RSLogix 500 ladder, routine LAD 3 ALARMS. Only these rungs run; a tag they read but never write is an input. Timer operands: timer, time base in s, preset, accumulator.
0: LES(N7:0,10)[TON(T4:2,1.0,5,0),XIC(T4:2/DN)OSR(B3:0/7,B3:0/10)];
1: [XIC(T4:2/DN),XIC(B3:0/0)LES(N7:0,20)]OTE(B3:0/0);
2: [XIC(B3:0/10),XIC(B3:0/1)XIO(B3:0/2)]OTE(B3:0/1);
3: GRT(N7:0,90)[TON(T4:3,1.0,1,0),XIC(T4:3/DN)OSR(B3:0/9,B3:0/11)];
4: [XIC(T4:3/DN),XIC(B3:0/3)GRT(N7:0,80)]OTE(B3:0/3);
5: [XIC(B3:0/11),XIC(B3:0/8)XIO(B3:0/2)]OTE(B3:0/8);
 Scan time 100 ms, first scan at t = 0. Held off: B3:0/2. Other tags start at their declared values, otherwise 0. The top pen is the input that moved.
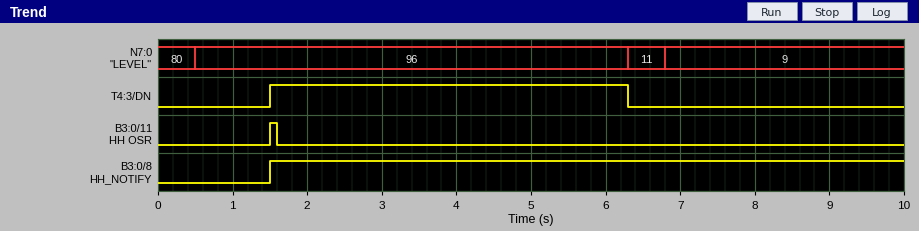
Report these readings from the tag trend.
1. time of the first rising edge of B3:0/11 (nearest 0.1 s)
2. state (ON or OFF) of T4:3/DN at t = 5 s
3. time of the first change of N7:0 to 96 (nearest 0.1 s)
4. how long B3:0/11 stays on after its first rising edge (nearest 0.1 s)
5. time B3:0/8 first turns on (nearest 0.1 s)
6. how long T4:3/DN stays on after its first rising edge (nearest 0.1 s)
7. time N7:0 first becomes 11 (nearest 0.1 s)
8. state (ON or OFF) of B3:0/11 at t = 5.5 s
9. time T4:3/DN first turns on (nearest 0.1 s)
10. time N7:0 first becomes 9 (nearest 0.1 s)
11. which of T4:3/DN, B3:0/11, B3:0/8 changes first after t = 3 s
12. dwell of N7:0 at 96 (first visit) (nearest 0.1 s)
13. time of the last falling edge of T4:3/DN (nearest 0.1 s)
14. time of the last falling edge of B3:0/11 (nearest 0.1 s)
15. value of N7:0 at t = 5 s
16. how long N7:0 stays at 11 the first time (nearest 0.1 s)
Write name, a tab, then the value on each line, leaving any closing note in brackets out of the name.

time of the first rising edge of B3:0/11	1.5 s
state (ON or OFF) of T4:3/DN at t = 5 s	ON
time of the first change of N7:0 to 96	0.5 s
how long B3:0/11 stays on after its first rising edge	0.1 s
time B3:0/8 first turns on	1.5 s
how long T4:3/DN stays on after its first rising edge	4.8 s
time N7:0 first becomes 11	6.3 s
state (ON or OFF) of B3:0/11 at t = 5.5 s	OFF
time T4:3/DN first turns on	1.5 s
time N7:0 first becomes 9	6.8 s
which of T4:3/DN, B3:0/11, B3:0/8 changes first after t = 3 s	T4:3/DN
dwell of N7:0 at 96 (first visit)	5.8 s
time of the last falling edge of T4:3/DN	6.3 s
time of the last falling edge of B3:0/11	1.6 s
value of N7:0 at t = 5 s	96
how long N7:0 stays at 11 the first time	0.5 s
